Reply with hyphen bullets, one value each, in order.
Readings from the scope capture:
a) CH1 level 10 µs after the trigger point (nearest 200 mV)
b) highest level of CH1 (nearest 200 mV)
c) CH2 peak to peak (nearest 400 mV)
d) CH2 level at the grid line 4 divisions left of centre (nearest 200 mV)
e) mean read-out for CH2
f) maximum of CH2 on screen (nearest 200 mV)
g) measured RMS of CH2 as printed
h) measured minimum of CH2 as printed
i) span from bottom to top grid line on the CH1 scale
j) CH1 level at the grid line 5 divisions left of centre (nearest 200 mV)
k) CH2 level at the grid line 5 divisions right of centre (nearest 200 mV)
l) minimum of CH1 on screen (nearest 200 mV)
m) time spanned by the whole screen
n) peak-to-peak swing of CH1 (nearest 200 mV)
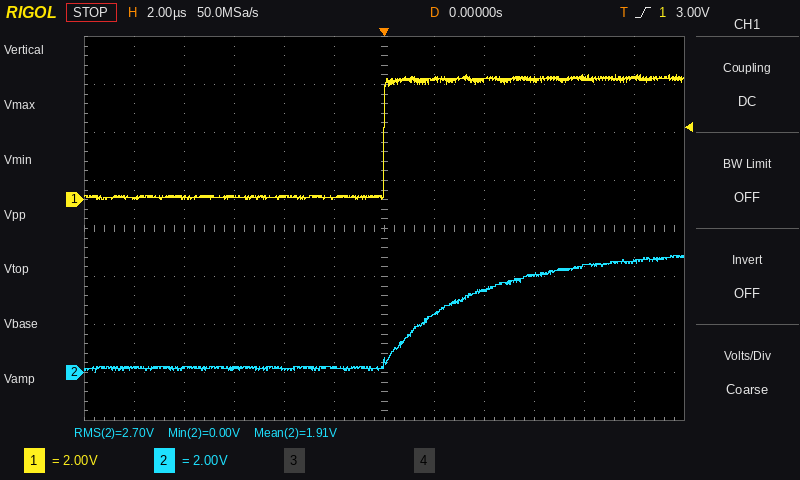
- 5.0 V
- 5.2 V
- 4.8 V
- 200 mV
- 1.91 V
- 4.8 V
- 2.70 V
- 0.00 V
- 16 V
- 0.0 V
- 4.6 V
- 0.0 V
- 24 µs
- 5.2 V
